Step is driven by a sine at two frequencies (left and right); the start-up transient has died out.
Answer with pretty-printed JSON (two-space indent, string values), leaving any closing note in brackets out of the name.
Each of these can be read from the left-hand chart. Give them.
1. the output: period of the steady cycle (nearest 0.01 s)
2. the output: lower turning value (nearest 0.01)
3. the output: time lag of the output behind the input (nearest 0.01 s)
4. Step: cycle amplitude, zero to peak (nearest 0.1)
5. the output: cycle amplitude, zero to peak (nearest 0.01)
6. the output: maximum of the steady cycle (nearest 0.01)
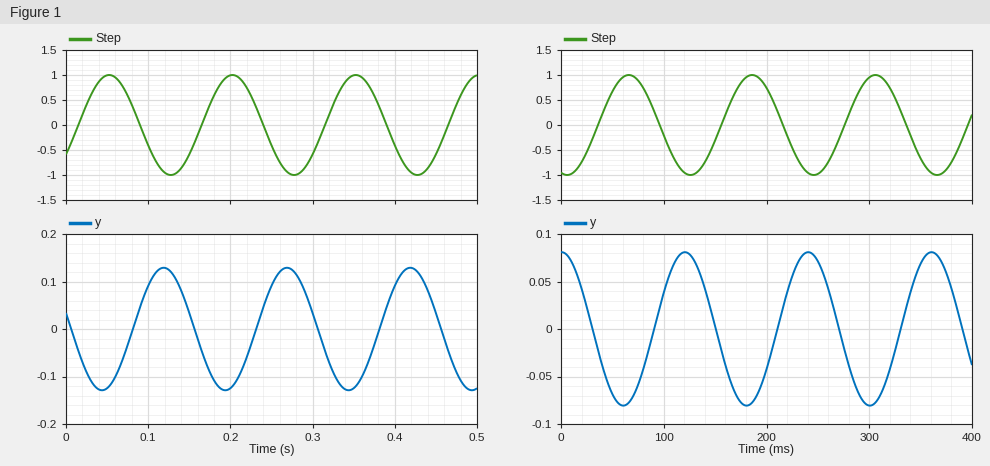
{
  "the output: period of the steady cycle": "0.15 s",
  "the output: lower turning value": "-0.13",
  "the output: time lag of the output behind the input": "0.07 s",
  "Step: cycle amplitude, zero to peak": "1.0",
  "the output: cycle amplitude, zero to peak": "0.13",
  "the output: maximum of the steady cycle": "0.13"
}
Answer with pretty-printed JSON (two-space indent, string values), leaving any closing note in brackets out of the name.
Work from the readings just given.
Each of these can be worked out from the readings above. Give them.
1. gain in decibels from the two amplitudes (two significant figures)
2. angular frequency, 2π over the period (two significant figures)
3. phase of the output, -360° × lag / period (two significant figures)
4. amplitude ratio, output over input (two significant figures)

{
  "gain in decibels from the two amplitudes": "-18 dB",
  "angular frequency, 2π over the period": "42 rad/s",
  "phase of the output, -360° × lag / period": "-170°",
  "amplitude ratio, output over input": "0.13"
}
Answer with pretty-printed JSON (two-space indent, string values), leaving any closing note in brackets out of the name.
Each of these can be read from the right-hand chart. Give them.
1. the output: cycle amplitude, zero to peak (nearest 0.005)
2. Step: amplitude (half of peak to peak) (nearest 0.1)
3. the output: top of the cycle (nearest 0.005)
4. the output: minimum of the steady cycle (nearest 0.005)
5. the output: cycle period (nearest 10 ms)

{
  "the output: cycle amplitude, zero to peak": "0.080",
  "Step: amplitude (half of peak to peak)": "1.0",
  "the output: top of the cycle": "0.080",
  "the output: minimum of the steady cycle": "-0.080",
  "the output: cycle period": "120 ms"
}
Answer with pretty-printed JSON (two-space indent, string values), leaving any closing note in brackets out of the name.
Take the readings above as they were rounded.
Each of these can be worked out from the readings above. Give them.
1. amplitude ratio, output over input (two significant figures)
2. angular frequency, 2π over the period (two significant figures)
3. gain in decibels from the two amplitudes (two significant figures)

{
  "amplitude ratio, output over input": "0.080",
  "angular frequency, 2π over the period": "0.052 rad/ms",
  "gain in decibels from the two amplitudes": "-22 dB"
}
